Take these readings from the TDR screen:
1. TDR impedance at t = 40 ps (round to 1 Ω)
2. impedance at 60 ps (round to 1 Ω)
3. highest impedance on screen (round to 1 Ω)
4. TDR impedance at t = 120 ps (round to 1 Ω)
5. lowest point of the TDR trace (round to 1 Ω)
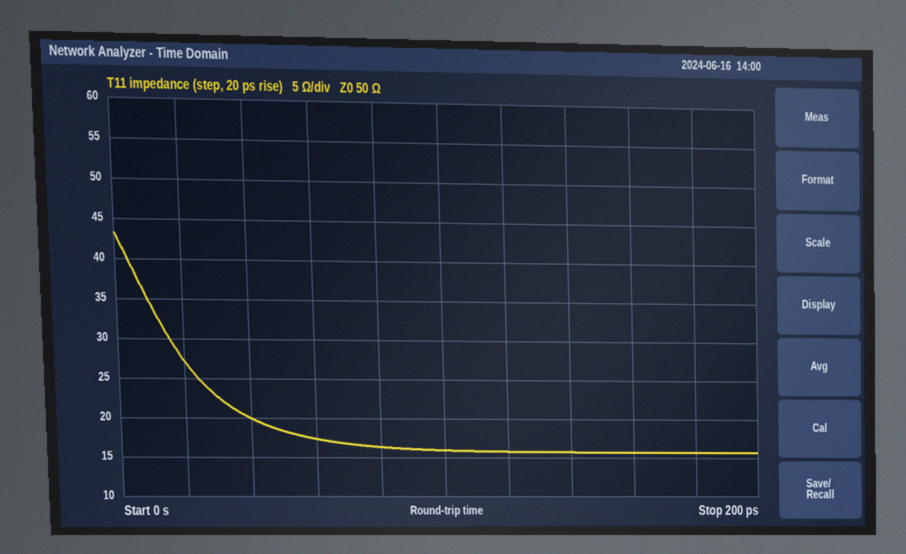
20 Ω
17 Ω
43 Ω
16 Ω
16 Ω
